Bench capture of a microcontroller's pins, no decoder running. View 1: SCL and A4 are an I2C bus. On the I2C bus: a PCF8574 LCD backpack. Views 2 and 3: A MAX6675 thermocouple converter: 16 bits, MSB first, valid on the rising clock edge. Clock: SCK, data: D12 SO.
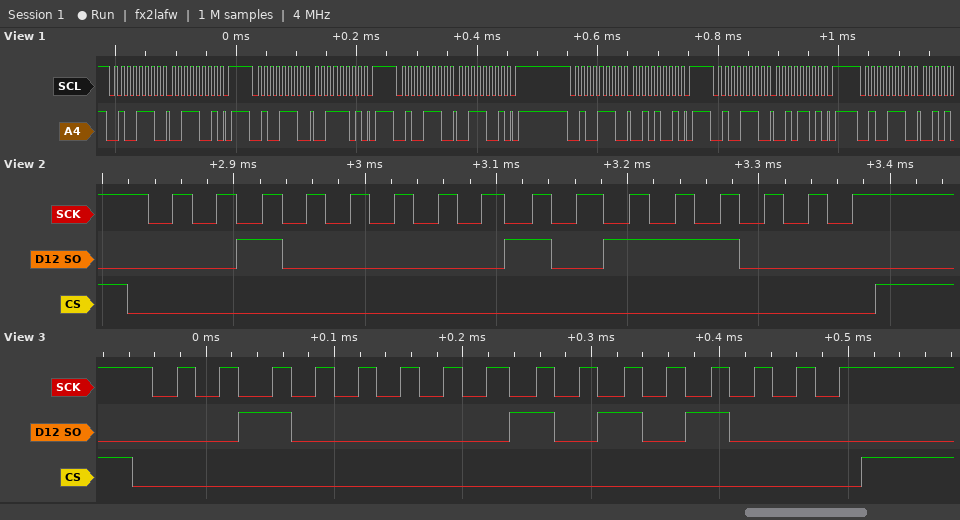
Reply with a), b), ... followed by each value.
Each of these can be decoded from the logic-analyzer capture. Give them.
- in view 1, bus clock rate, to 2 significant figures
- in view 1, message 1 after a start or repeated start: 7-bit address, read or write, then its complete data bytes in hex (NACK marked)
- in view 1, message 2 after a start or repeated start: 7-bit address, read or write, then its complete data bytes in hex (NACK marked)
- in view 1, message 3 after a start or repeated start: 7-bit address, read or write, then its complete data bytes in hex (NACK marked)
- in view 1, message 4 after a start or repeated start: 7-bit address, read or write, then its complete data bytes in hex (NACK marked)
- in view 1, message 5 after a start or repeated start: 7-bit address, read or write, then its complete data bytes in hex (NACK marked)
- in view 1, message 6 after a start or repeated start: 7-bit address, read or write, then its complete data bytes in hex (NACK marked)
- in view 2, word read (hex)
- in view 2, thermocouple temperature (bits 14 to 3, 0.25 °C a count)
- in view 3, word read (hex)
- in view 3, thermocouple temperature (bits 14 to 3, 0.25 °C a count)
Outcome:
a) 100 kHz
b) 0x27 write: 39
c) 0x27 write: 3D
d) 0x27 write: 39
e) 0x27 write: 29
f) 0x27 write: 2D
g) 0x27 write
h) 0x20B8
i) 261.75 °C
j) 0x20A8
k) 261.25 °C
